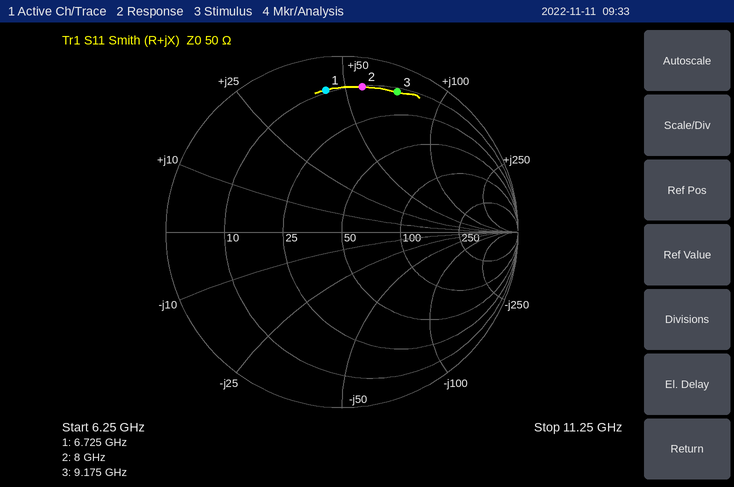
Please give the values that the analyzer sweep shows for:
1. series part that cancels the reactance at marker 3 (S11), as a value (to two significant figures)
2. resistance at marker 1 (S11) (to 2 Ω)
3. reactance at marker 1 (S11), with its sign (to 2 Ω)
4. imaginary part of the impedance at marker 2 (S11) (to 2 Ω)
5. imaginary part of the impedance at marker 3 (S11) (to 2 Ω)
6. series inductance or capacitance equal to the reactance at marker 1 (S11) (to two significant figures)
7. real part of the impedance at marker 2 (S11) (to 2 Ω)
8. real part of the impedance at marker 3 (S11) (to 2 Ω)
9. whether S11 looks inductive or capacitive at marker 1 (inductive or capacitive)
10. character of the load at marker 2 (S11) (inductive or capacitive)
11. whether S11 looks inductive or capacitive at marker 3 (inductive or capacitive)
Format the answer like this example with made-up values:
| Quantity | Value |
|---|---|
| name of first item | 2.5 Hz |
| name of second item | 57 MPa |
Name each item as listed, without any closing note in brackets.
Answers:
| Quantity | Value |
|---|---|
| series part that cancels the reactance at marker 3 (S11), as a value | 240 fF |
| resistance at marker 1 (S11) | 10 Ω |
| reactance at marker 1 (S11), with its sign | +44 Ω |
| imaginary part of the impedance at marker 2 (S11) | +56 Ω |
| imaginary part of the impedance at marker 3 (S11) | +72 Ω |
| series inductance or capacitance equal to the reactance at marker 1 (S11) | 1.0 nH |
| real part of the impedance at marker 2 (S11) | 10 Ω |
| real part of the impedance at marker 3 (S11) | 12 Ω |
| whether S11 looks inductive or capacitive at marker 1 | inductive |
| character of the load at marker 2 (S11) | inductive |
| whether S11 looks inductive or capacitive at marker 3 | inductive |
